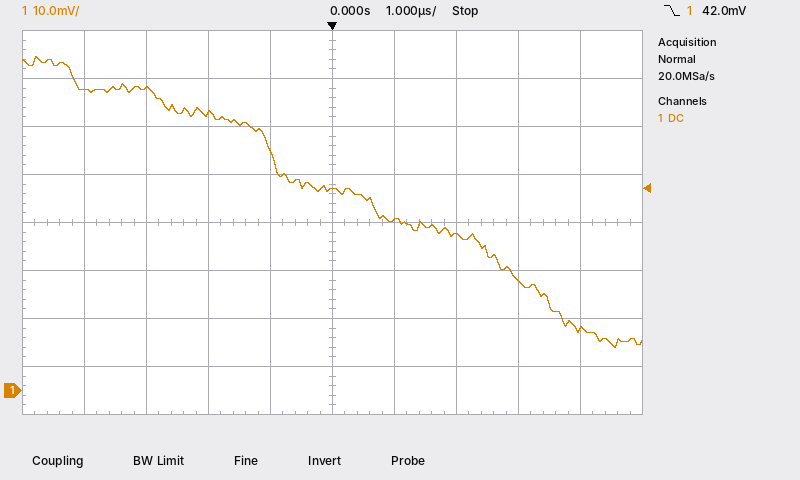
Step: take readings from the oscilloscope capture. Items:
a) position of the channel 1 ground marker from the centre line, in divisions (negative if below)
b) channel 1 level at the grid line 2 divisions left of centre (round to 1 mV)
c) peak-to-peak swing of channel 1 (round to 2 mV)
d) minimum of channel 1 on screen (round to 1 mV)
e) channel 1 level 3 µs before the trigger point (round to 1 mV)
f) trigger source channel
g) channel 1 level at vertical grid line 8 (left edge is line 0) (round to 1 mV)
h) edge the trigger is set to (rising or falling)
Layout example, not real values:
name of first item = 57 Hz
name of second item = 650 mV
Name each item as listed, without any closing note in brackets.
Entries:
position of the channel 1 ground marker from the centre line, in divisions = -3.5 div
channel 1 level at the grid line 2 divisions left of centre = 58 mV
peak-to-peak swing of channel 1 = 60 mV
minimum of channel 1 on screen = 9 mV
channel 1 level 3 µs before the trigger point = 63 mV
trigger source channel = channel 1
channel 1 level at vertical grid line 8 (left edge is line 0) = 23 mV
edge the trigger is set to = falling
